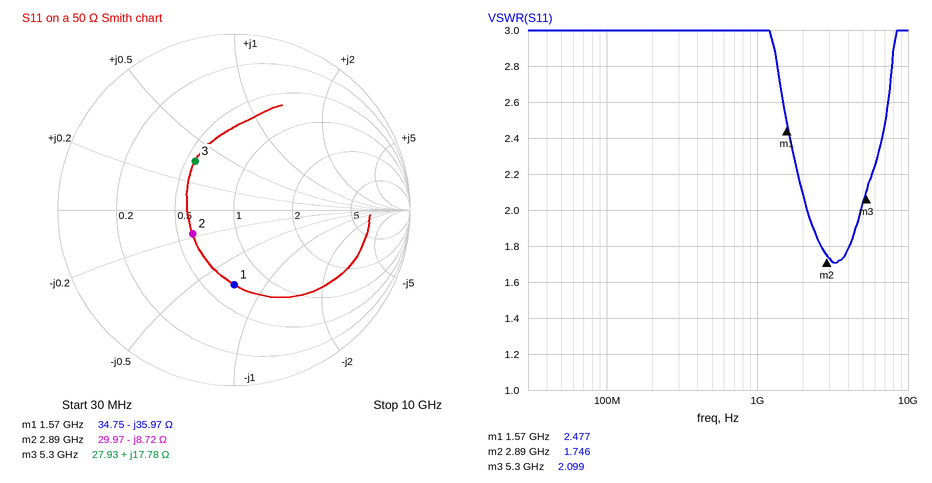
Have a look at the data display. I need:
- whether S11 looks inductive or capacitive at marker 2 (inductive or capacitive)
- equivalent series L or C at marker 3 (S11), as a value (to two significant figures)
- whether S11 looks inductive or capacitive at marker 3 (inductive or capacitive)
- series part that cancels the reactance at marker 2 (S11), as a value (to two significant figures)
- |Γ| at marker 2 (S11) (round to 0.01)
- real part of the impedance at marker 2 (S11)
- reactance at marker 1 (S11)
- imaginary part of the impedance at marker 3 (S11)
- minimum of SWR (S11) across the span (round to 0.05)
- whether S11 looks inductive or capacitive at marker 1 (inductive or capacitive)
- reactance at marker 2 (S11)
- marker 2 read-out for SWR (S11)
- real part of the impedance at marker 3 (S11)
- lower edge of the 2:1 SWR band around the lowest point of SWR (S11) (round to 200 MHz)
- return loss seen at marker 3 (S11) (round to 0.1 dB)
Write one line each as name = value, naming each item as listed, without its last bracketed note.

whether S11 looks inductive or capacitive at marker 2 = capacitive
equivalent series L or C at marker 3 (S11), as a value = 530 pH
whether S11 looks inductive or capacitive at marker 3 = inductive
series part that cancels the reactance at marker 2 (S11), as a value = 480 pH
|Γ| at marker 2 (S11) = 0.27
real part of the impedance at marker 2 = 29.97 Ω
reactance at marker 1 = -35.97 Ω
imaginary part of the impedance at marker 3 = +17.78 Ω
minimum of SWR (S11) across the span = 1.70
whether S11 looks inductive or capacitive at marker 1 = capacitive
reactance at marker 2 = -8.72 Ω
marker 2 read-out for SWR = 1.746
real part of the impedance at marker 3 = 27.93 Ω
lower edge of the 2:1 SWR band around the lowest point of SWR (S11) = 2.2 GHz
return loss seen at marker 3 (S11) = 9.0 dB
